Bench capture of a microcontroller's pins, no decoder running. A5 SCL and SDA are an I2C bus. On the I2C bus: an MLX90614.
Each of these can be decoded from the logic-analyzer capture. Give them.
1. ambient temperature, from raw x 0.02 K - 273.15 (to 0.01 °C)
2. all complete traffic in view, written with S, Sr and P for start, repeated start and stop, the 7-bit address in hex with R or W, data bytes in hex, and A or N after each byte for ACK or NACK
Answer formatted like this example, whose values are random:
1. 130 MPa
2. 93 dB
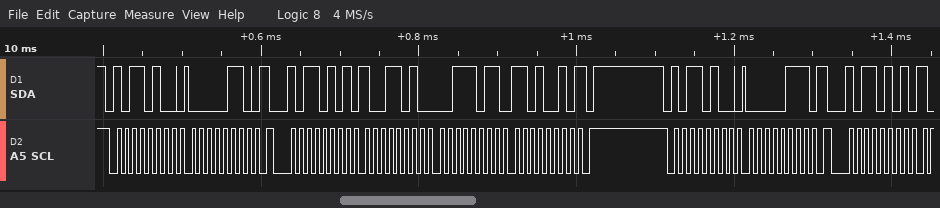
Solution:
1. 32.01 °C
2. S 5AW A 06 A Sr 5AR A 9A A 3B A D2 N P S 5AW A 07 A Sr 5AR A
